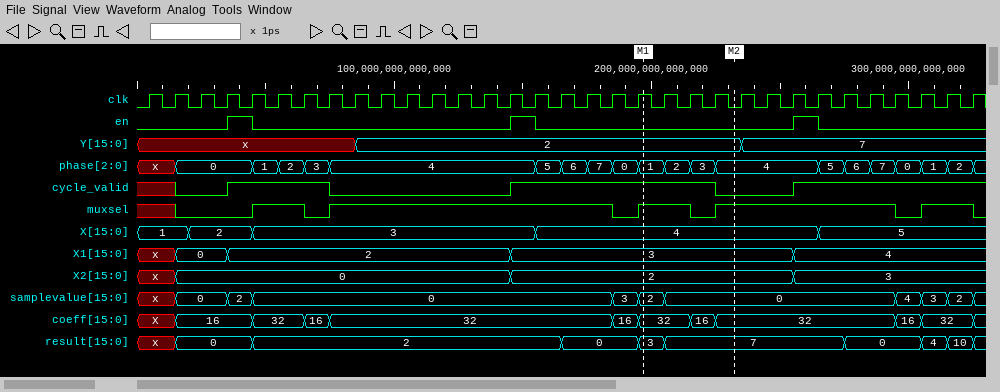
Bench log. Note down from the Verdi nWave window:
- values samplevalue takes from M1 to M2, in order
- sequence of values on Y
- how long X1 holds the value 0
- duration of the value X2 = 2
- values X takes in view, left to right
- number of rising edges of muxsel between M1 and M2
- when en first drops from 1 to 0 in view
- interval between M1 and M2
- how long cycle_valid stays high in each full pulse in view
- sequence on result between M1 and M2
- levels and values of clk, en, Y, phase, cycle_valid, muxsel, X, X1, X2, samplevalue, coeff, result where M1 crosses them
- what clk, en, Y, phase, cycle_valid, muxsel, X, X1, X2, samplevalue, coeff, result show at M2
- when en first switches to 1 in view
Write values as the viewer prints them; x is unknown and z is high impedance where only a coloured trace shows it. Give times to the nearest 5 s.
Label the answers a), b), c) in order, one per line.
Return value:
a) 2, 0
b) x, 2, 7
c) 20 s
d) 110 s
e) 1, 2, 3, 4, 5
f) 1
g) 45 s
h) 35 s
i) 40 s, 80 s
j) 3, 7
k) clk=1, en=0, Y=2, phase=1, cycle_valid=1, muxsel=1, X=4, X1=3, X2=2, samplevalue=2, coeff=32, result=3
l) clk=0, en=0, Y=2, phase=4, cycle_valid=0, muxsel=1, X=4, X1=3, X2=2, samplevalue=0, coeff=32, result=7
m) 35 s
